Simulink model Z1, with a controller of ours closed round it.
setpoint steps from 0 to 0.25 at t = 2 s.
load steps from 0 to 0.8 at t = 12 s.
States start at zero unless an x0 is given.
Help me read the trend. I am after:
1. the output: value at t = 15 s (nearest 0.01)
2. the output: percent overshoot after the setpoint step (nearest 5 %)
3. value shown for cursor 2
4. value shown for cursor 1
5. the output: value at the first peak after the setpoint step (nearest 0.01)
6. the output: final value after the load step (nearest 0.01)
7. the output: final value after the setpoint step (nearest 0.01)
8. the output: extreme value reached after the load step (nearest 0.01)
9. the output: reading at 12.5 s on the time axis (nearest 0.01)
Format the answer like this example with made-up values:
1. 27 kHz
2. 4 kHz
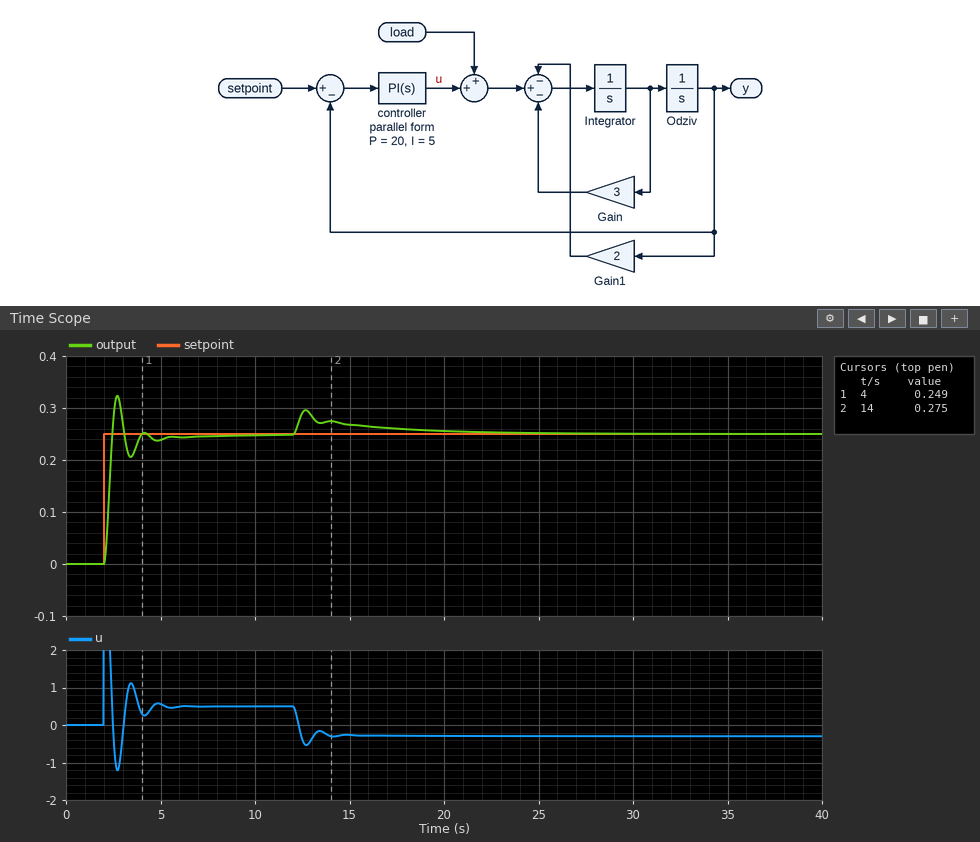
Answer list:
1. 0.27
2. 30 %
3. 0.275
4. 0.249
5. 0.32
6. 0.25
7. 0.25
8. 0.30
9. 0.29
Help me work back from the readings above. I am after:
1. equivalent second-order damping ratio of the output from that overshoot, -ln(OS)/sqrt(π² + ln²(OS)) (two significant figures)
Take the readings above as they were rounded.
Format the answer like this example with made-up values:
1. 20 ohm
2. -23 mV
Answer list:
1. 0.36
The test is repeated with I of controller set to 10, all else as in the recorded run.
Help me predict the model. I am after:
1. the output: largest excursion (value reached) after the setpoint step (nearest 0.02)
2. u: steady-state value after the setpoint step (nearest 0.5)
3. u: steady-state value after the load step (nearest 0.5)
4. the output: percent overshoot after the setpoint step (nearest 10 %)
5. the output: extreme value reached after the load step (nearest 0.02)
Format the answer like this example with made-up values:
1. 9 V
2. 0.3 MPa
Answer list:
1. 0.34
2. 0.5
3. -0.5
4. 40 %
5. 0.30
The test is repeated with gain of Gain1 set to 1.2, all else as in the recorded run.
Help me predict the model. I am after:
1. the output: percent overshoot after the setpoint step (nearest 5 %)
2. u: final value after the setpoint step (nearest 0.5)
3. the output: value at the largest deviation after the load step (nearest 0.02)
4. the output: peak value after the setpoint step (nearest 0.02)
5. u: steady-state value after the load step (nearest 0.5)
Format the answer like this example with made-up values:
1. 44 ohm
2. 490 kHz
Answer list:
1. 35 %
2. 0.5
3. 0.30
4. 0.34
5. -0.5
